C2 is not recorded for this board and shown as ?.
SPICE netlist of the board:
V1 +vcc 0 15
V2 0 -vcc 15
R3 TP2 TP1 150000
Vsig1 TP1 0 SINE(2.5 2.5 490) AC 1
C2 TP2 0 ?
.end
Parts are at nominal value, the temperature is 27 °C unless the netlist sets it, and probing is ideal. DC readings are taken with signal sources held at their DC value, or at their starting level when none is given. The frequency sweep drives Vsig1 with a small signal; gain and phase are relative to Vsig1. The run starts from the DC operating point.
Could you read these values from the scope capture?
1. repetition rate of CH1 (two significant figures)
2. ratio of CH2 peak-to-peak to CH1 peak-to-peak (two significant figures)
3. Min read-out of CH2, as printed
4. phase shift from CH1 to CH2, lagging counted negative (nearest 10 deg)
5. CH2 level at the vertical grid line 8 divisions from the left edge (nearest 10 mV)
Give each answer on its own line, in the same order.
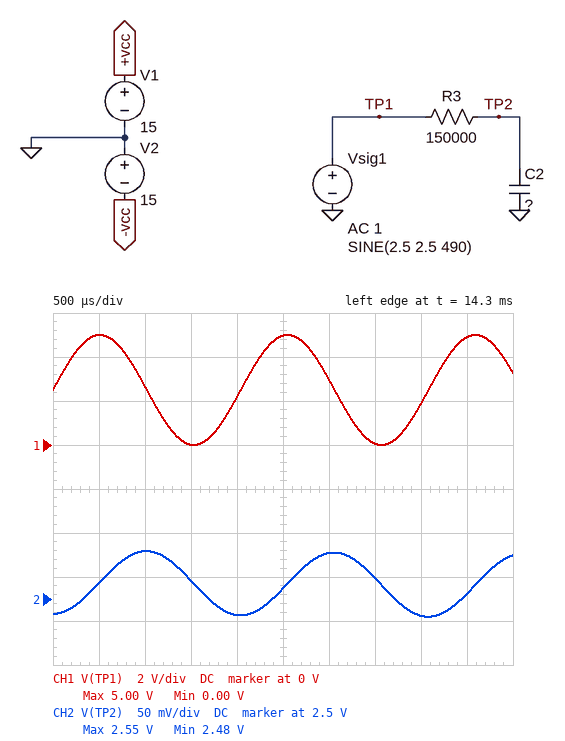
490 Hz
0.015
2.48 V
-90 deg
2.48 V
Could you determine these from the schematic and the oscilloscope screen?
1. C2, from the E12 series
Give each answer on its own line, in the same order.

150 nF
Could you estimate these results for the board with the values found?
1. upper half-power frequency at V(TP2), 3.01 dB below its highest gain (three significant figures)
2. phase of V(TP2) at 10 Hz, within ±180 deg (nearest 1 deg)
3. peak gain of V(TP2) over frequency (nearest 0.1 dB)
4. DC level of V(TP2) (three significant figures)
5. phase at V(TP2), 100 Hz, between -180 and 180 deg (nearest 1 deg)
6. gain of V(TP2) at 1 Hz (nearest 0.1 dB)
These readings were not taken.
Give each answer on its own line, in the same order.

7.07 Hz
-55 deg
0 dB
2.50 V
-86 deg
-0.1 dB
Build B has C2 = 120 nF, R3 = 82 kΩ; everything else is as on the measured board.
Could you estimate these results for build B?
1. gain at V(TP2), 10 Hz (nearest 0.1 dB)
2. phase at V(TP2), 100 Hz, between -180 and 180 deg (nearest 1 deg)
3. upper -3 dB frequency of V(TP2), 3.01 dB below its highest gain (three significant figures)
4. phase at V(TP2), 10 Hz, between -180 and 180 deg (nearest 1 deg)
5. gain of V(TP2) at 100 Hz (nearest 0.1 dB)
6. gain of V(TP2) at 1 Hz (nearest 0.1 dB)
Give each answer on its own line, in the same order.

-1.4 dB
-81 deg
16.2 Hz
-32 deg
-15.9 dB
0 dB
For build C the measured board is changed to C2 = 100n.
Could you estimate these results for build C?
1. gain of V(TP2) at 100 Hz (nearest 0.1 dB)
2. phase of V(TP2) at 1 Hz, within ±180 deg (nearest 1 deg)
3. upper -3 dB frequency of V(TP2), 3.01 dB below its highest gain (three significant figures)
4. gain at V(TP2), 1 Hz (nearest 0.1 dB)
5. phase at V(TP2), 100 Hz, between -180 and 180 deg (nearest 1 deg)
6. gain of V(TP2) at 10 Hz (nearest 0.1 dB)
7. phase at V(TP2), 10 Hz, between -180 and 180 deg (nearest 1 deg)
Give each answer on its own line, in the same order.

-19.5 dB
-5 deg
10.6 Hz
0 dB
-84 deg
-2.8 dB
-43 deg
